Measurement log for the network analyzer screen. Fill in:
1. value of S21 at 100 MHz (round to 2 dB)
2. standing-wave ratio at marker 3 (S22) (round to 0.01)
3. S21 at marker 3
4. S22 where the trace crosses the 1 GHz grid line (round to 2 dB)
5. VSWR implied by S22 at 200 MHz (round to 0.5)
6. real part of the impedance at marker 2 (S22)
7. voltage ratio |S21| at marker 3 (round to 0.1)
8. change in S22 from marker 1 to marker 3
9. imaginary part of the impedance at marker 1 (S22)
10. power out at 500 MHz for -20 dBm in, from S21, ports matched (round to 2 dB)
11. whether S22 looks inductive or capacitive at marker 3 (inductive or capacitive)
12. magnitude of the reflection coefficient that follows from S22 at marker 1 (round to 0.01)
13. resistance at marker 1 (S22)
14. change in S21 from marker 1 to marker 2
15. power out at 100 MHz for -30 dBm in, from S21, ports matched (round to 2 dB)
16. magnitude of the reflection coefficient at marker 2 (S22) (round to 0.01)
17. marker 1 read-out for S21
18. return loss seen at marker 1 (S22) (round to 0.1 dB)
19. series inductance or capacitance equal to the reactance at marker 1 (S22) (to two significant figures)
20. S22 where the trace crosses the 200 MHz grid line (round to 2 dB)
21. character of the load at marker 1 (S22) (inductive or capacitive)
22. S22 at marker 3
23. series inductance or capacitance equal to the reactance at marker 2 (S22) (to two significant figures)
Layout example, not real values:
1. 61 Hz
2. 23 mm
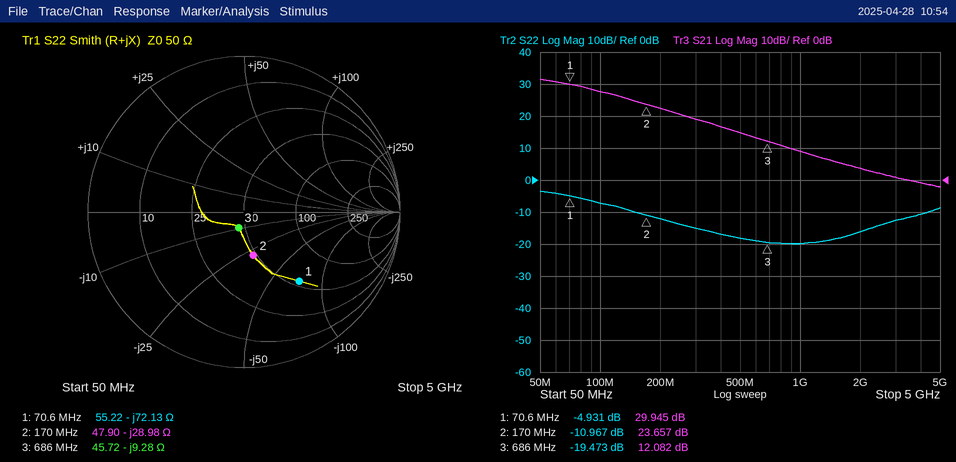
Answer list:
1. 28 dB
2. 1.24
3. 12.082 dB
4. -20 dB
5. 1.5
6. 47.90 Ω
7. 4.0
8. -14.542 dB
9. -72.13 Ω
10. -6 dBm
11. capacitive
12. 0.57
13. 55.22 Ω
14. -6.288 dB
15. -2 dBm
16. 0.28
17. 29.945 dB
18. 4.9 dB
19. 31 pF
20. -12 dB
21. capacitive
22. -19.473 dB
23. 32 pF
